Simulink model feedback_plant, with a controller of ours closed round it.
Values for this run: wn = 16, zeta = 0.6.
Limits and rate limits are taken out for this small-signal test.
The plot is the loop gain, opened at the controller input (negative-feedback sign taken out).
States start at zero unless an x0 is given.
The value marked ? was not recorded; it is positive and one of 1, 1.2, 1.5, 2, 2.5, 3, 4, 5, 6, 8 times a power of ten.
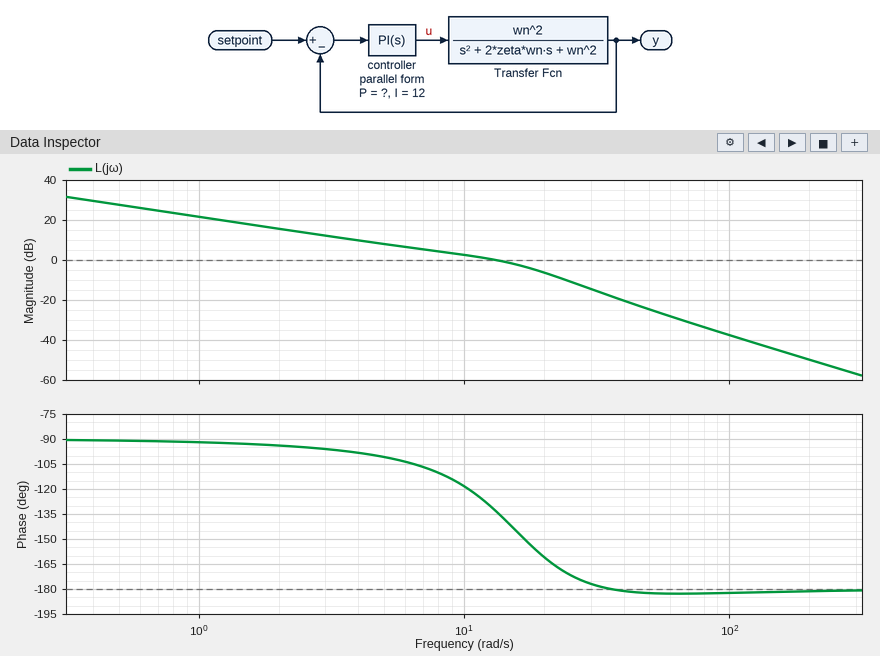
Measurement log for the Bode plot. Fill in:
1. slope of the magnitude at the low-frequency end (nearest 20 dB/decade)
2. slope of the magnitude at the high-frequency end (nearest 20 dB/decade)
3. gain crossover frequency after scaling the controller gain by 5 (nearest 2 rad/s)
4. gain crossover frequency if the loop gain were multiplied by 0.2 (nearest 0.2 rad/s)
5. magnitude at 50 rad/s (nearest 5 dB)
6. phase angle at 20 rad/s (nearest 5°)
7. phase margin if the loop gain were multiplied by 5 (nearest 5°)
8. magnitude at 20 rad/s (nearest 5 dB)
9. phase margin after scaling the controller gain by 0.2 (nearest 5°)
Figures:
-20 dB/decade
-40 dB/decade
30 rad/s
2.4 rad/s
-25 dB
-160°
5°
-5 dB
85°
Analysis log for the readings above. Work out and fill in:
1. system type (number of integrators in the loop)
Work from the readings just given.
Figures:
1
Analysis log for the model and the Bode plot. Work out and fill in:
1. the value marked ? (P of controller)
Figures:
0.5
